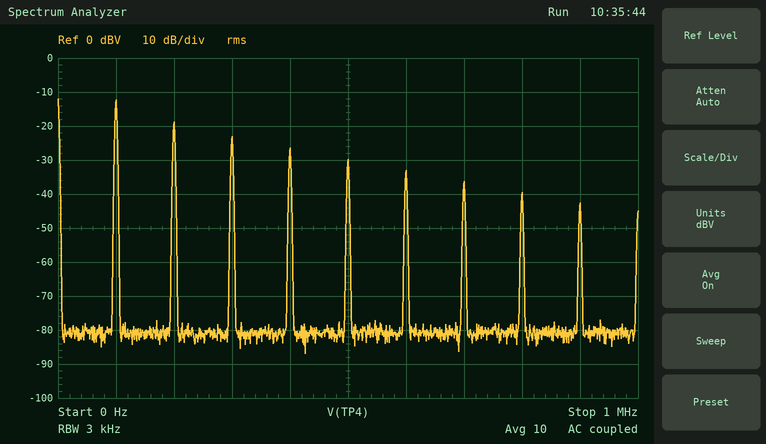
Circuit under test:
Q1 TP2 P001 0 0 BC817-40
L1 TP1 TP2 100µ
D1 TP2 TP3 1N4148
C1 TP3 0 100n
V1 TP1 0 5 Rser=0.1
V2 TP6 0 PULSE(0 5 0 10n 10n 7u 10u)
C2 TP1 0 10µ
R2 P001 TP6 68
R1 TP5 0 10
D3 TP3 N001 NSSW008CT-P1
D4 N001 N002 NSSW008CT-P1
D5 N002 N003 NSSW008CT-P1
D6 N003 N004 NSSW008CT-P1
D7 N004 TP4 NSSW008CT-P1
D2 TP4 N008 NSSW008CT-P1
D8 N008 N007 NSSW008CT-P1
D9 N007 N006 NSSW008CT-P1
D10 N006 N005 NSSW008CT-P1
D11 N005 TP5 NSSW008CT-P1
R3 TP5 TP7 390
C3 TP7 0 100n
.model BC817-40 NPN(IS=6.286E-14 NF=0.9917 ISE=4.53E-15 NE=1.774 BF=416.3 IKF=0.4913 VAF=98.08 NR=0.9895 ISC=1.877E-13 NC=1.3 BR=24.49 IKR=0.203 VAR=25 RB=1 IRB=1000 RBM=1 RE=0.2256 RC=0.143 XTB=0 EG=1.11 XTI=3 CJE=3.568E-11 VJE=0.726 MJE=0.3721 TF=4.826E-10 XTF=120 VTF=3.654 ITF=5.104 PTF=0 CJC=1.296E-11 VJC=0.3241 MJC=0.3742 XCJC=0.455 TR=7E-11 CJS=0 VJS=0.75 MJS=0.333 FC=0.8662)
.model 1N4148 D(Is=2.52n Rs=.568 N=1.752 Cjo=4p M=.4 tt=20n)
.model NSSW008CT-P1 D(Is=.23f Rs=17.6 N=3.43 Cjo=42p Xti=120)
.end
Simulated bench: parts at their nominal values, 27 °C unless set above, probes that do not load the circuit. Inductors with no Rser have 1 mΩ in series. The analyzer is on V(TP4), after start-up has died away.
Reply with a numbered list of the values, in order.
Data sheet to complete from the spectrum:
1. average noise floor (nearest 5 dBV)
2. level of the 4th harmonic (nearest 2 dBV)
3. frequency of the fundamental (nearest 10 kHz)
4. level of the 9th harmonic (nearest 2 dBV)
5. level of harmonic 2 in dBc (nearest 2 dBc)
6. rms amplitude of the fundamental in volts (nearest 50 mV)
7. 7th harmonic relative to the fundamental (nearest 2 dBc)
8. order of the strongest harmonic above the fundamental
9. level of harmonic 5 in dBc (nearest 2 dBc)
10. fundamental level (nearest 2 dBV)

1. -80 dBV
2. -26 dBV
3. 100 kHz
4. -42 dBV
5. -6 dBc
6. 250 mV
7. -24 dBc
8. 2
9. -18 dBc
10. -12 dBV
